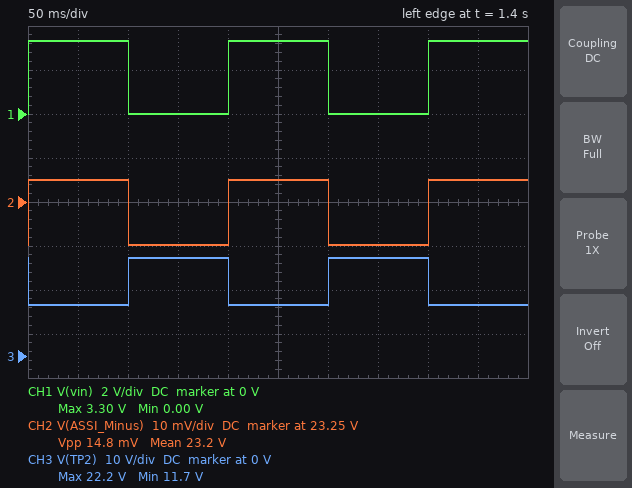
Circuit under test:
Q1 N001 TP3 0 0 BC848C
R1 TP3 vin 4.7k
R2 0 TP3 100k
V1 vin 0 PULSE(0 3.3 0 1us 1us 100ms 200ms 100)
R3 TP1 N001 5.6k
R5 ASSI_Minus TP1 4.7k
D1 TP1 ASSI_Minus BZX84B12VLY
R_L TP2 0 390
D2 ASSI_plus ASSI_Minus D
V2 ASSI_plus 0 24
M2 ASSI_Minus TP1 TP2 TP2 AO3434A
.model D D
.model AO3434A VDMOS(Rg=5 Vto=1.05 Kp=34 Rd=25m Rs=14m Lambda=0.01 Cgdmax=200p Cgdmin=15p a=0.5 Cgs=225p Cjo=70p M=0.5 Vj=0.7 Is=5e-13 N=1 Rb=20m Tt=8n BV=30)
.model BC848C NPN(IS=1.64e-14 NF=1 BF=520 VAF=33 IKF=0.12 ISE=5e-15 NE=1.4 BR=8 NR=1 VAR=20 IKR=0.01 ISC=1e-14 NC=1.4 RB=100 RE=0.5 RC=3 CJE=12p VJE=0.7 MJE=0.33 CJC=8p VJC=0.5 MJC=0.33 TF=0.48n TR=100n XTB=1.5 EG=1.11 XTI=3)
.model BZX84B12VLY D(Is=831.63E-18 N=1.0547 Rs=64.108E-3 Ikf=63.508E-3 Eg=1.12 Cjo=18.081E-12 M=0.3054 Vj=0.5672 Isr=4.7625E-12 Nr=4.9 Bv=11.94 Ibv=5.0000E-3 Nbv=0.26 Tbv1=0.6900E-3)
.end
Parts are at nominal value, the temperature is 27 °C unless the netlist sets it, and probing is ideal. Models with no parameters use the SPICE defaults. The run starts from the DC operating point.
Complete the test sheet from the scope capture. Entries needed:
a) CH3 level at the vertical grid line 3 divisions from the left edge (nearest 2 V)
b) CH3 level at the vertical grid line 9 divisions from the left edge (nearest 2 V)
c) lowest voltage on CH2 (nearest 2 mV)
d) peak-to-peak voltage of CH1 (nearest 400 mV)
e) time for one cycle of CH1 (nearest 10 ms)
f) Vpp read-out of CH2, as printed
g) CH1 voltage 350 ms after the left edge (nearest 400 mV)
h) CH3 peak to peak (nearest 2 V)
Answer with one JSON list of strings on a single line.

["22 V", "12 V", "23.240 V", "3.2 V", "200 ms", "14.8 mV", "0 V", "10 V"]
